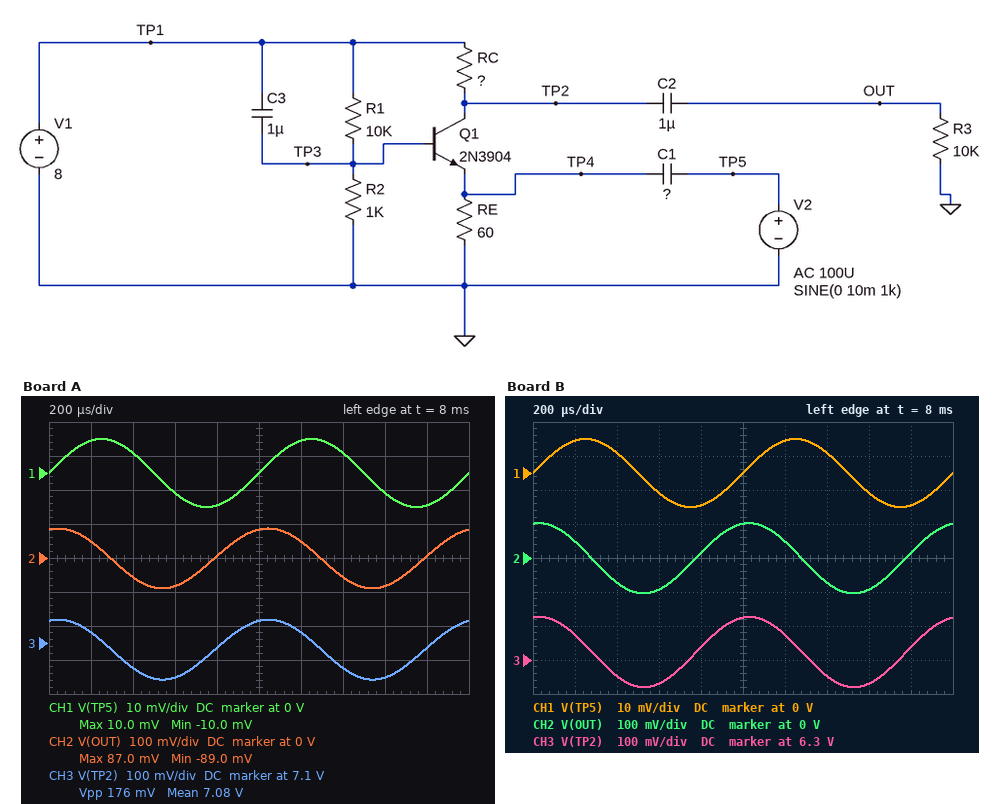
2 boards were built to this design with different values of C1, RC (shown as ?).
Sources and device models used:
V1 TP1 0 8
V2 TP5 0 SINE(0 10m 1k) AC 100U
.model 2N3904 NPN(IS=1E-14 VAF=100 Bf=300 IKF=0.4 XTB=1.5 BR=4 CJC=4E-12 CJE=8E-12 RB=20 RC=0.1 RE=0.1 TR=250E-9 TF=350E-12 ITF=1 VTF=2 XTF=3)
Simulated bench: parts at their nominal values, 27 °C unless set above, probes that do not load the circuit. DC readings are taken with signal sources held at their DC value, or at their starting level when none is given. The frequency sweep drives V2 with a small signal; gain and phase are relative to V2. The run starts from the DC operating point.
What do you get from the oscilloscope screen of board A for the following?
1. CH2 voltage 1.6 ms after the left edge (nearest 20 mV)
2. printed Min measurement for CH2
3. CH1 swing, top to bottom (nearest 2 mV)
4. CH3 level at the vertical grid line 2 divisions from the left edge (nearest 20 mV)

-80 mV
-89.0 mV
20 mV
7.02 V
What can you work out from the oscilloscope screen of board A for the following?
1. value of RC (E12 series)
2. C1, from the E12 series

820 Ω
2.7 µF
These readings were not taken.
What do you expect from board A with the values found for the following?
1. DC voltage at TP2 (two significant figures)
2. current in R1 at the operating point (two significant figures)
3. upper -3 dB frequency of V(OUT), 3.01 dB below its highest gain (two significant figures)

7.1 V
730 µA
53 MHz
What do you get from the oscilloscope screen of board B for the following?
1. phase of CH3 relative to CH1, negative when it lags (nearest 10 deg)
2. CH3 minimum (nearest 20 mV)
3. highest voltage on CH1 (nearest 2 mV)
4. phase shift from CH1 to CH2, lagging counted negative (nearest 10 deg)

80 deg
6.22 V
10 mV
80 deg
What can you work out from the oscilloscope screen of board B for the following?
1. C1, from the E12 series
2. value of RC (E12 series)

1.8 µF
1.5 kΩ
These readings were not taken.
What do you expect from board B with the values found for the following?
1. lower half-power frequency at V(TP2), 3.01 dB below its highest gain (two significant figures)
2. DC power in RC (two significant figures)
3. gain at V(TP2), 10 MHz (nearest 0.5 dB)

5.2 kHz
1.9 mW
34.5 dB
